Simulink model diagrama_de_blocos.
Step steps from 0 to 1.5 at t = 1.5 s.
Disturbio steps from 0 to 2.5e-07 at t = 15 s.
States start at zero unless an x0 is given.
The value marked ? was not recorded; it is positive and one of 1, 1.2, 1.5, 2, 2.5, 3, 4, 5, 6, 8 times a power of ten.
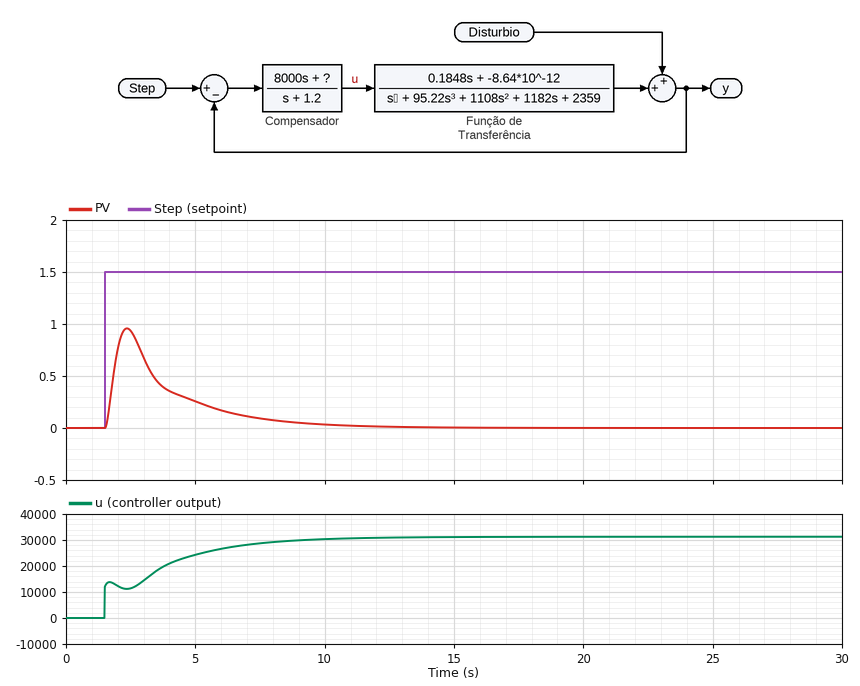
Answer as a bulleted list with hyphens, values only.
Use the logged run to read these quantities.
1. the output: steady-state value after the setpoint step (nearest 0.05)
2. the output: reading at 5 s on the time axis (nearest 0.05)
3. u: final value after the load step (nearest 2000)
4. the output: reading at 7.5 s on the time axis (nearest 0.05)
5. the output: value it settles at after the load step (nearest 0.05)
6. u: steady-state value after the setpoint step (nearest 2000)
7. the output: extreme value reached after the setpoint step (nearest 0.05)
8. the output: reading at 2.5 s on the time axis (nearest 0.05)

- 0.00
- 0.25
- 32000
- 0.10
- 0.00
- 32000
- 0.95
- 0.95
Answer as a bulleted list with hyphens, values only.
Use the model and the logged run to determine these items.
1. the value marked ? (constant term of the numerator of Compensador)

- 25000
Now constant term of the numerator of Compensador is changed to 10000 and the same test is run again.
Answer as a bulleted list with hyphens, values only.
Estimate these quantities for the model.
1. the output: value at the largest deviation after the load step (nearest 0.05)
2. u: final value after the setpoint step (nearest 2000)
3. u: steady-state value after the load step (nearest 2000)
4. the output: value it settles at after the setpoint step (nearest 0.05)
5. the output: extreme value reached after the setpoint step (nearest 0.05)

- 0.00
- 12000
- 12000
- 0.00
- 0.65
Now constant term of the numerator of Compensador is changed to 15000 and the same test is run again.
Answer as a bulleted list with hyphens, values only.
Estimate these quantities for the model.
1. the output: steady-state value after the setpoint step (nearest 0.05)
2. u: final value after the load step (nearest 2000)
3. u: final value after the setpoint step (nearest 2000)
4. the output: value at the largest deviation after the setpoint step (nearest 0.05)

- 0.00
- 18000
- 18000
- 0.75
